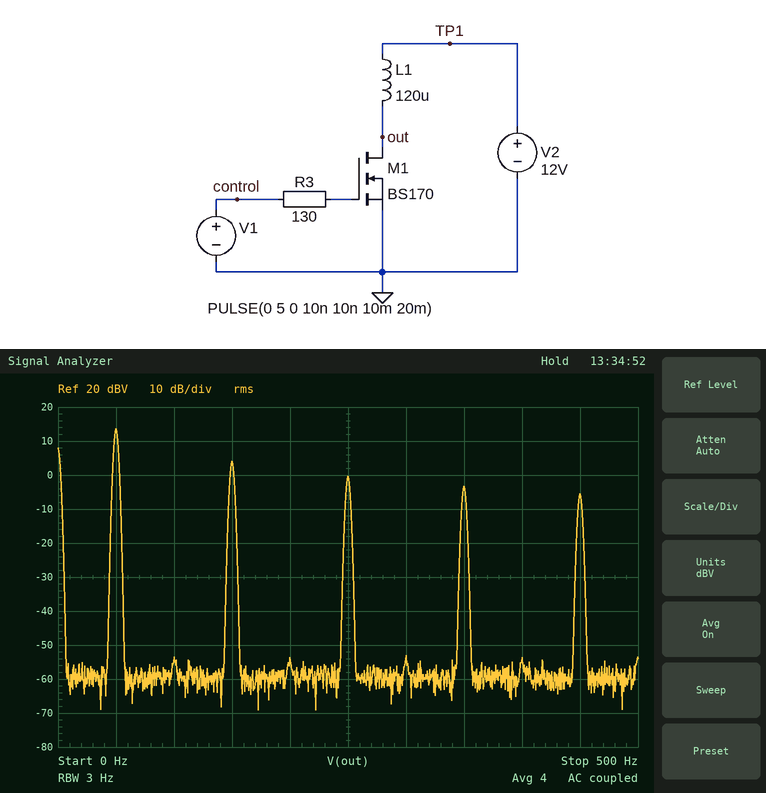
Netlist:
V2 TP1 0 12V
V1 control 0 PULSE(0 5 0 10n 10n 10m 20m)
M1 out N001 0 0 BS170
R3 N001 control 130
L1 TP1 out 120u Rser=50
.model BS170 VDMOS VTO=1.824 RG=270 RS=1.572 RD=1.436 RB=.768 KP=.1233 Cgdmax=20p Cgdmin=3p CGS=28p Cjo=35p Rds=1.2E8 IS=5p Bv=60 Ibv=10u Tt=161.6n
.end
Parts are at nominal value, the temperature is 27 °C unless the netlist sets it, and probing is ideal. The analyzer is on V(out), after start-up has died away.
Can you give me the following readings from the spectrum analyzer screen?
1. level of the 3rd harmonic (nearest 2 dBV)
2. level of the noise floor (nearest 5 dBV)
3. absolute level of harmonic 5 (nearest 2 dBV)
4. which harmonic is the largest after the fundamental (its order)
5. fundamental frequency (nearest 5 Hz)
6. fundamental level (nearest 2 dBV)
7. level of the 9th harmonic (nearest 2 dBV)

4 dBV
-60 dBV
0 dBV
3
50 Hz
14 dBV
-6 dBV
